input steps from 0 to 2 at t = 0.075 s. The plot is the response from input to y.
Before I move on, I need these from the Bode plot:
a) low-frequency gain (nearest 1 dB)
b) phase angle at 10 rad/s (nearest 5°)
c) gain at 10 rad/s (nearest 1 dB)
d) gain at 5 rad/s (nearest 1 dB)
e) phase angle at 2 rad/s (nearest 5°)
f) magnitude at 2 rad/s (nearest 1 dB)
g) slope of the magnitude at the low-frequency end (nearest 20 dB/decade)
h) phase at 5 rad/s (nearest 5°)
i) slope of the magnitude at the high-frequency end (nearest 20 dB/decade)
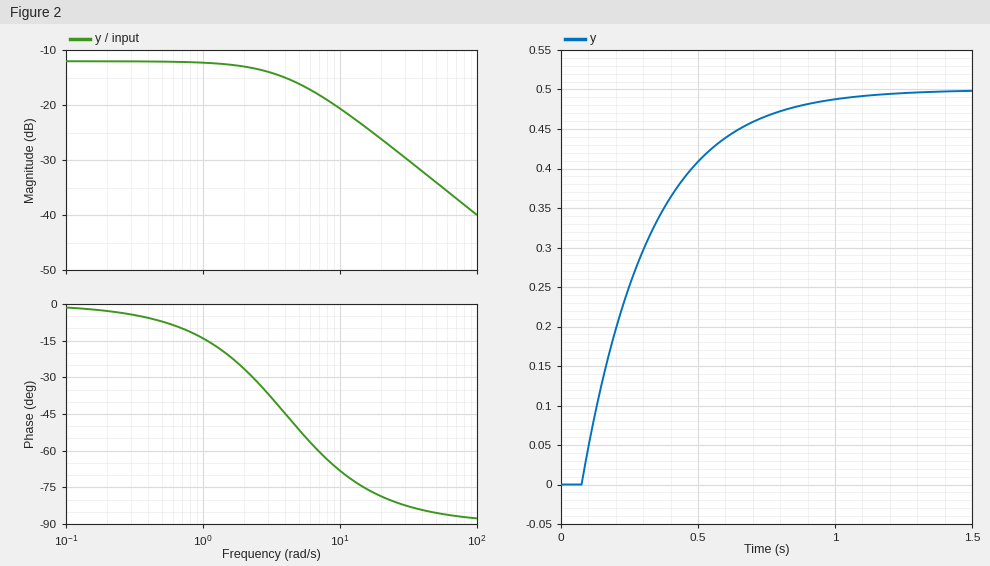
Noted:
-12 dB
-70°
-21 dB
-16 dB
-25°
-13 dB
0 dB/decade
-50°
-20 dB/decade
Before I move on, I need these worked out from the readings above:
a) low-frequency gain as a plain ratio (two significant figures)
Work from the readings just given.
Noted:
0.25
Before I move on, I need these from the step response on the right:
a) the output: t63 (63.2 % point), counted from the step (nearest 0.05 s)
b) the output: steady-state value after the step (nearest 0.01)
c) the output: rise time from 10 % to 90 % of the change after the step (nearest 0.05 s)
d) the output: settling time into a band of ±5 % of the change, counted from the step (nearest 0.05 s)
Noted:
0.25 s
0.50
0.55 s
0.75 s
